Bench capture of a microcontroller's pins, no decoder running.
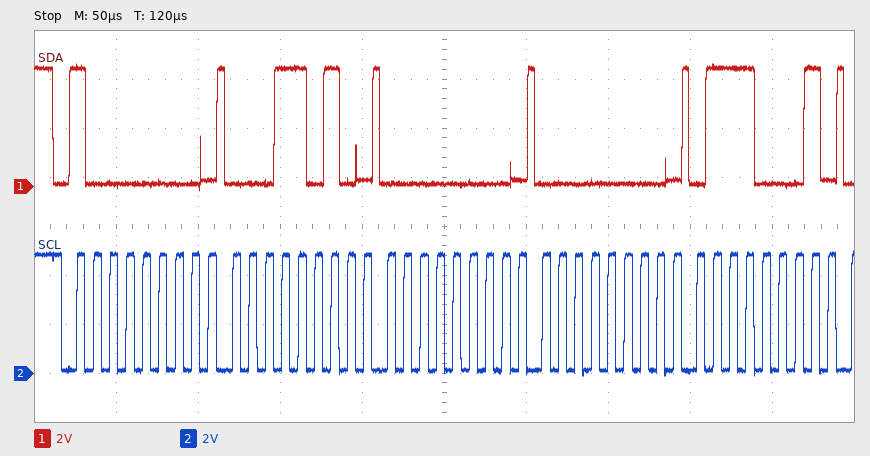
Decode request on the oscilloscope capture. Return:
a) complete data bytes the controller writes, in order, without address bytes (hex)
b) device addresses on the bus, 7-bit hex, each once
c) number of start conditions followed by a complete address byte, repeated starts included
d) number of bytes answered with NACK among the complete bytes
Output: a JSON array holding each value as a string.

["1A 00 00 71", "0x40", "1", "0"]
